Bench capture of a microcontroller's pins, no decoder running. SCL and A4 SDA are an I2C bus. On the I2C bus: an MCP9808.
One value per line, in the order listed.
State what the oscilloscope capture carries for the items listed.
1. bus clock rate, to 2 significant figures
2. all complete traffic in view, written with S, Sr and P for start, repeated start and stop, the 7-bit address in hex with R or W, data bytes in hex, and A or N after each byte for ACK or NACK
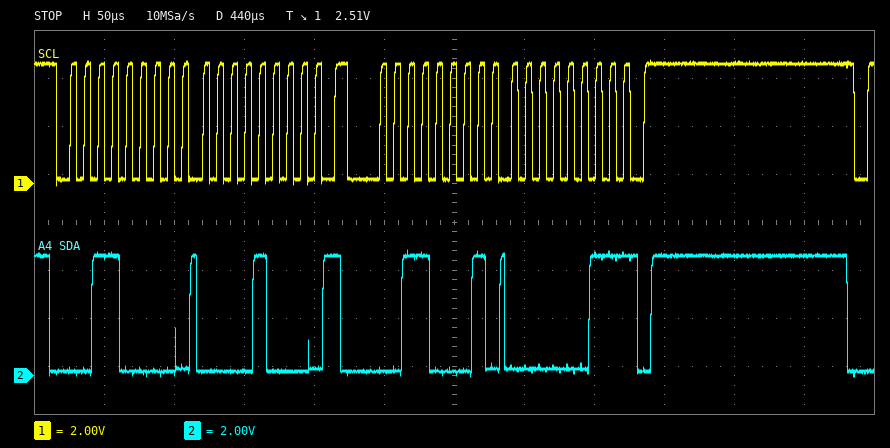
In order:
100 kHz
S 18W A 08 A Sr 18R A 03 N P
